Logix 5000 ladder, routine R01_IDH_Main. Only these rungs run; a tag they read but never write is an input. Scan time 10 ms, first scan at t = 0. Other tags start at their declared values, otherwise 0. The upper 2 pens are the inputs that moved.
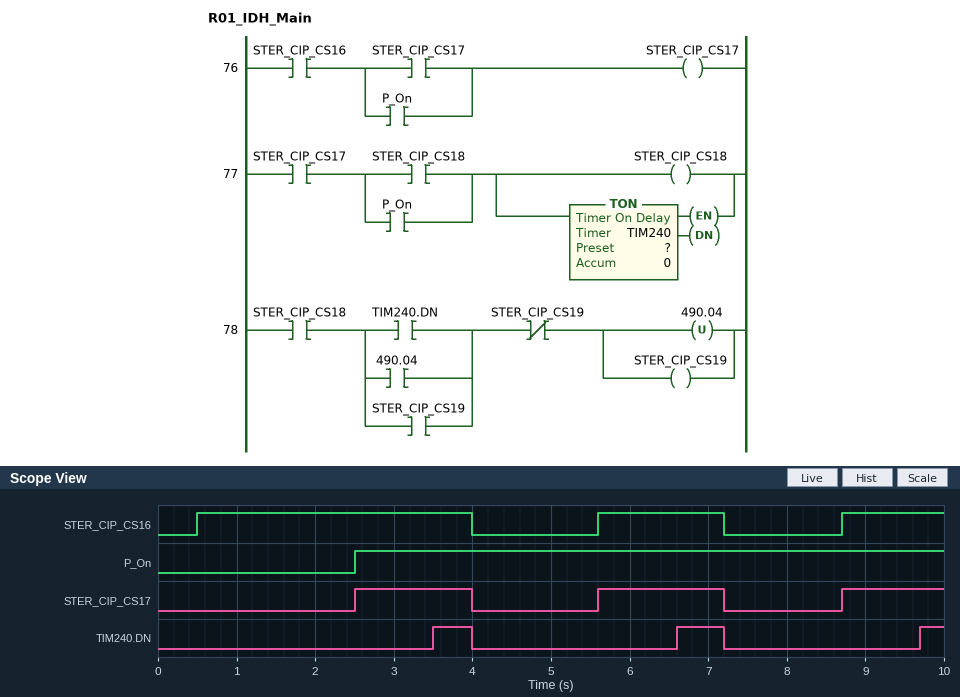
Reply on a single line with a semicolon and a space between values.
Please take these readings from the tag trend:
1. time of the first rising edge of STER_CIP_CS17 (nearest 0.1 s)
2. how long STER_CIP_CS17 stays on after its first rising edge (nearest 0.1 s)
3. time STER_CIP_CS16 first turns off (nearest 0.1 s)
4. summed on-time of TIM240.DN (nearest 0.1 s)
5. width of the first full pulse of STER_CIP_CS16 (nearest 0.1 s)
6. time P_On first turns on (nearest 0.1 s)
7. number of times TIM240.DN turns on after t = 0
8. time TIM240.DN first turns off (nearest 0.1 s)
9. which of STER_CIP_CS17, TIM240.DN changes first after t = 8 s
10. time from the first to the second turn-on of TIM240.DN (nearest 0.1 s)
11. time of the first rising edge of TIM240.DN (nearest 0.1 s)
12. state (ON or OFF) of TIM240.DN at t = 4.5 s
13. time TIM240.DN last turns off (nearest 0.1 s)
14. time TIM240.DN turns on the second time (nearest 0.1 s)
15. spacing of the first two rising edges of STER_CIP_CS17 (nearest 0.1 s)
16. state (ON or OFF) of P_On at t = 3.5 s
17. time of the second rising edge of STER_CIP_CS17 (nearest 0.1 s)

2.5 s; 1.5 s; 4.0 s; 1.4 s; 3.5 s; 2.5 s; 3; 4.0 s; STER_CIP_CS17; 3.1 s; 3.5 s; OFF; 7.2 s; 6.6 s; 3.1 s; ON; 5.6 s
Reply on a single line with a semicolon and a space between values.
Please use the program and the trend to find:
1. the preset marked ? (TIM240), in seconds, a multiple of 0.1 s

1.0 s
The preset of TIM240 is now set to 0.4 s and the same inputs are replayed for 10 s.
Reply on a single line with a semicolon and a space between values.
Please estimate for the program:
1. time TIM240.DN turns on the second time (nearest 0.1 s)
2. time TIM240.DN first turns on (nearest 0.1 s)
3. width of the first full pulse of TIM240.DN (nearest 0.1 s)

6.0 s; 2.9 s; 1.1 s
